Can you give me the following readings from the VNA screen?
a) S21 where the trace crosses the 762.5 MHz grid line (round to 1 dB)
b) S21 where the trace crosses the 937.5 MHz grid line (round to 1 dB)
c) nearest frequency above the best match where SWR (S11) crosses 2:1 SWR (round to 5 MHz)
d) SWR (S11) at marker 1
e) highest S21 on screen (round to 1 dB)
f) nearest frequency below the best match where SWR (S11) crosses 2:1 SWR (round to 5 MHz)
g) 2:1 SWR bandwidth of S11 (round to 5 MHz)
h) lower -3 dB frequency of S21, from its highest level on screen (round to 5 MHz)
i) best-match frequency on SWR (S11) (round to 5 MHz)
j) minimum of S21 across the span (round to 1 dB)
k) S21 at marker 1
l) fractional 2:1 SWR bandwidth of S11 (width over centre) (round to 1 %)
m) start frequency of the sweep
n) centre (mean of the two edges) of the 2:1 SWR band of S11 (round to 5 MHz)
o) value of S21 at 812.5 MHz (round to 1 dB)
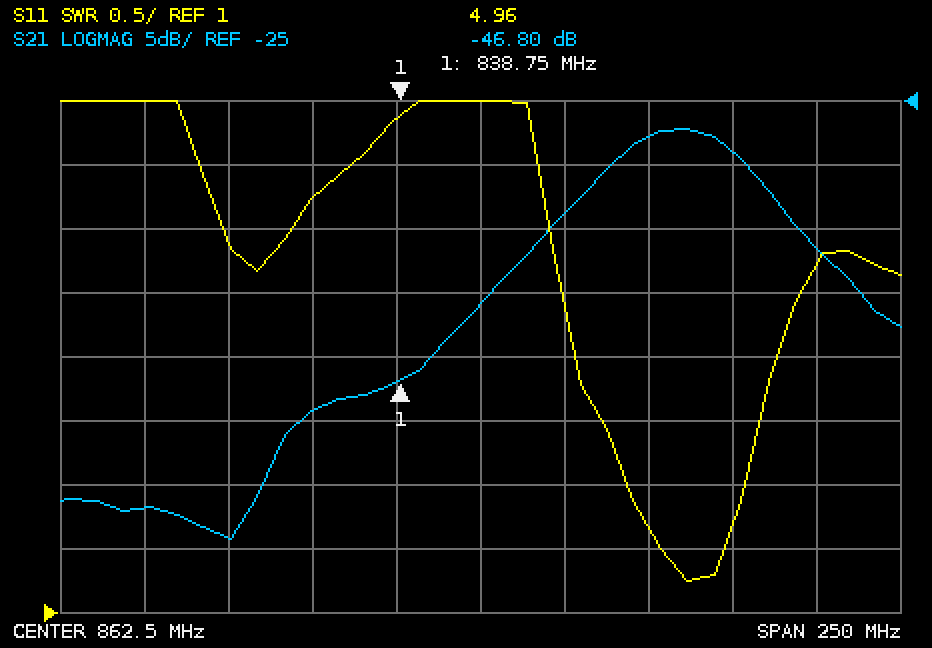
-57 dB
-29 dB
940 MHz
4.96
-27 dB
905 MHz
35 MHz
900 MHz
925 MHz
-59 dB
-46.80 dB
4 %
737.5 MHz
925 MHz
-49 dB
